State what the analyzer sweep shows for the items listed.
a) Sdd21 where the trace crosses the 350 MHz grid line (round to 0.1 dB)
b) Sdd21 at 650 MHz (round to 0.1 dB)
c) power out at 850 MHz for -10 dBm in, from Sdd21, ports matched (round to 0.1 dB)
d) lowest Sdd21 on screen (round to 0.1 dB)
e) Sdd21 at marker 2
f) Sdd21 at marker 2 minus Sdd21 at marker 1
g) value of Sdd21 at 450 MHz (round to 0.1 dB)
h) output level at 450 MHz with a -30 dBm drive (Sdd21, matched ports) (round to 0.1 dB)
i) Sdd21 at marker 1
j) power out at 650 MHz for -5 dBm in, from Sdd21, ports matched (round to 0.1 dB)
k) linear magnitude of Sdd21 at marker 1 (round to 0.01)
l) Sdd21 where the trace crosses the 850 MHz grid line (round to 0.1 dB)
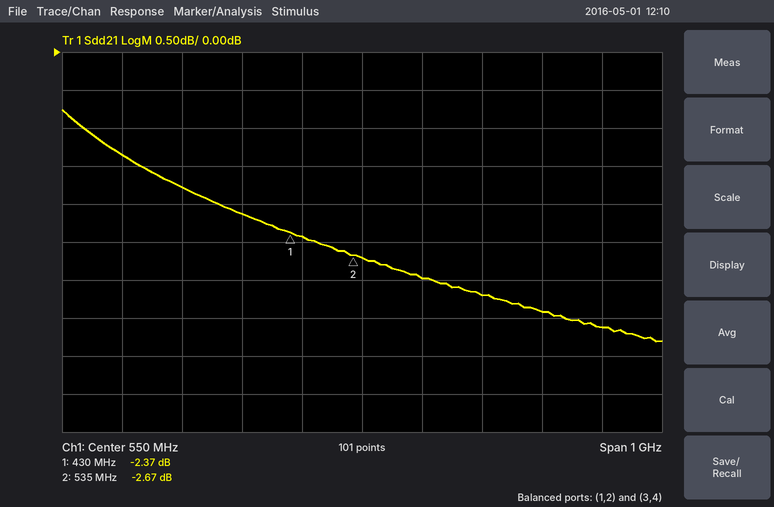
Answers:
-2.1 dB
-3.0 dB
-13.4 dBm
-3.8 dB
-2.67 dB
-0.30 dB
-2.4 dB
-32.4 dBm
-2.37 dB
-8.0 dBm
0.76
-3.4 dB
